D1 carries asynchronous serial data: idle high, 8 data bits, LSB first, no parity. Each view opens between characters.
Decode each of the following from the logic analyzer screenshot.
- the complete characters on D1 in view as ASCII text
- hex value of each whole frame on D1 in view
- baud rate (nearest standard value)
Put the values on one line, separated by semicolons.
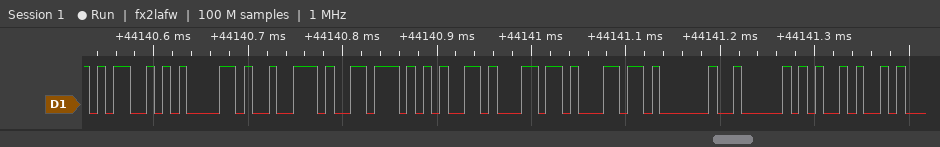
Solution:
"Marvell PJ"; 4D, 61, 72, 76, 65, 6C, 6C, 20, 50, 4A; 115200 baud
